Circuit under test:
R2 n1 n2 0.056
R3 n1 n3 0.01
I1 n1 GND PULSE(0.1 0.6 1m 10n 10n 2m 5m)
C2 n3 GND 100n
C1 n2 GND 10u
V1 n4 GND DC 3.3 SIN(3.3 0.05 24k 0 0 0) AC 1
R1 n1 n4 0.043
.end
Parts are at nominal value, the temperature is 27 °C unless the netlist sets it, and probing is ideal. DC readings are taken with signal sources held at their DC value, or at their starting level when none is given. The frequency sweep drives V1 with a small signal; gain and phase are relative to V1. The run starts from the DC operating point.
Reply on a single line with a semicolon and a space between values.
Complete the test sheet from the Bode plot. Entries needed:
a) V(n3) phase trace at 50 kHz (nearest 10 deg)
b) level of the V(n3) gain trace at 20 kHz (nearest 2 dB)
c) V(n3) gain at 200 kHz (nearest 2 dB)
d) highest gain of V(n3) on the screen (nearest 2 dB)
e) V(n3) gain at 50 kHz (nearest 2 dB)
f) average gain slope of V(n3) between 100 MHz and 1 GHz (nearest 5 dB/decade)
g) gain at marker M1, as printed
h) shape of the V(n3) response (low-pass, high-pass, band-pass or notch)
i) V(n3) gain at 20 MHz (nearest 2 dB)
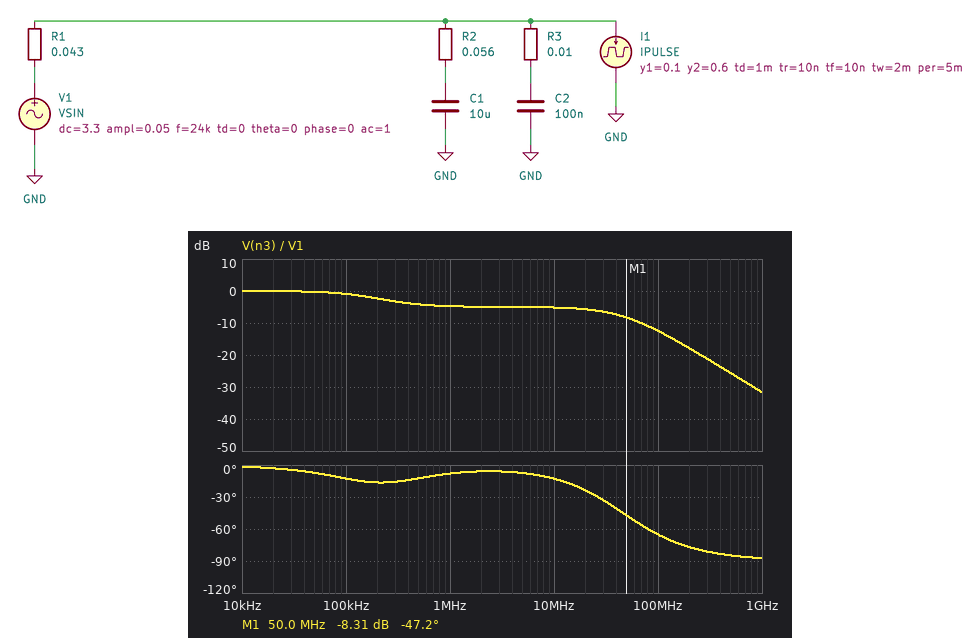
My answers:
-10 deg; 0 dB; -2 dB; 0 dB; 0 dB; -20 dB/decade; -8.31 dB; low-pass; -6 dB
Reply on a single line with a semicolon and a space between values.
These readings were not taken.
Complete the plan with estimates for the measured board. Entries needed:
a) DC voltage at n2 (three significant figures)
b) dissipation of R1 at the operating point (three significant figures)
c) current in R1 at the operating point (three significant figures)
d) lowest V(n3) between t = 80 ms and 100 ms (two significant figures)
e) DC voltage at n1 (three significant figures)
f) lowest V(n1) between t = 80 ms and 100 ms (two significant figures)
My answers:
3.30 V; 430 µW; 100 mA; 3.2 V; 3.30 V; 3.2 V
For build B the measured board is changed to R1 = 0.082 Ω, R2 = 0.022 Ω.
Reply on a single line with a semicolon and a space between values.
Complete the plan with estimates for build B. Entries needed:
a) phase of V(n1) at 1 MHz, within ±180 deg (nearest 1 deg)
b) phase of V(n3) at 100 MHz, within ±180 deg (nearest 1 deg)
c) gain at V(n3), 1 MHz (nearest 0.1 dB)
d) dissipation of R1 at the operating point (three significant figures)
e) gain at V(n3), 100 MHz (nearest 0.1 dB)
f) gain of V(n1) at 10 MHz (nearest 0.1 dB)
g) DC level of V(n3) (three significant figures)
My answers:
-28 deg; -60 deg; -11.8 dB; 820 µW; -19.5 dB; -13.6 dB; 3.29 V
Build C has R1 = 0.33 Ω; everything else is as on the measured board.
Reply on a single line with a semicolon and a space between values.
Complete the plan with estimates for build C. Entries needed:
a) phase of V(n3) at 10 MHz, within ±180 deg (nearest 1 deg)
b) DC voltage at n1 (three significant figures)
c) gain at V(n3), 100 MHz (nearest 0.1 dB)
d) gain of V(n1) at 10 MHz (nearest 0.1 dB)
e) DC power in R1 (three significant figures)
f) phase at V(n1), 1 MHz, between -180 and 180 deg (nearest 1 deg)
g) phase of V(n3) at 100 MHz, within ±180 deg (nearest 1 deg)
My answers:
-21 deg; 3.27 V; -28.3 dB; -17.3 dB; 3.30 mW; -15 deg; -75 deg
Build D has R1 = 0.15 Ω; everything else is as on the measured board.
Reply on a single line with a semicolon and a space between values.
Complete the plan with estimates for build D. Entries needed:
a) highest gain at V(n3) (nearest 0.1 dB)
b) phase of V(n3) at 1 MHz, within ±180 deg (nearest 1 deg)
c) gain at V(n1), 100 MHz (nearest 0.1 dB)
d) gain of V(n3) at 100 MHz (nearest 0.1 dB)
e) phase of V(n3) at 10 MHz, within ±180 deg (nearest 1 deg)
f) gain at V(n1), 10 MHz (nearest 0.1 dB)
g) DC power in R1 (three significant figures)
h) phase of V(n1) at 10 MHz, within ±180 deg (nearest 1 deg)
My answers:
0 dB; -13 deg; -20.4 dB; -21.8 dB; -19 deg; -11.8 dB; 1.50 mW; -15 deg
